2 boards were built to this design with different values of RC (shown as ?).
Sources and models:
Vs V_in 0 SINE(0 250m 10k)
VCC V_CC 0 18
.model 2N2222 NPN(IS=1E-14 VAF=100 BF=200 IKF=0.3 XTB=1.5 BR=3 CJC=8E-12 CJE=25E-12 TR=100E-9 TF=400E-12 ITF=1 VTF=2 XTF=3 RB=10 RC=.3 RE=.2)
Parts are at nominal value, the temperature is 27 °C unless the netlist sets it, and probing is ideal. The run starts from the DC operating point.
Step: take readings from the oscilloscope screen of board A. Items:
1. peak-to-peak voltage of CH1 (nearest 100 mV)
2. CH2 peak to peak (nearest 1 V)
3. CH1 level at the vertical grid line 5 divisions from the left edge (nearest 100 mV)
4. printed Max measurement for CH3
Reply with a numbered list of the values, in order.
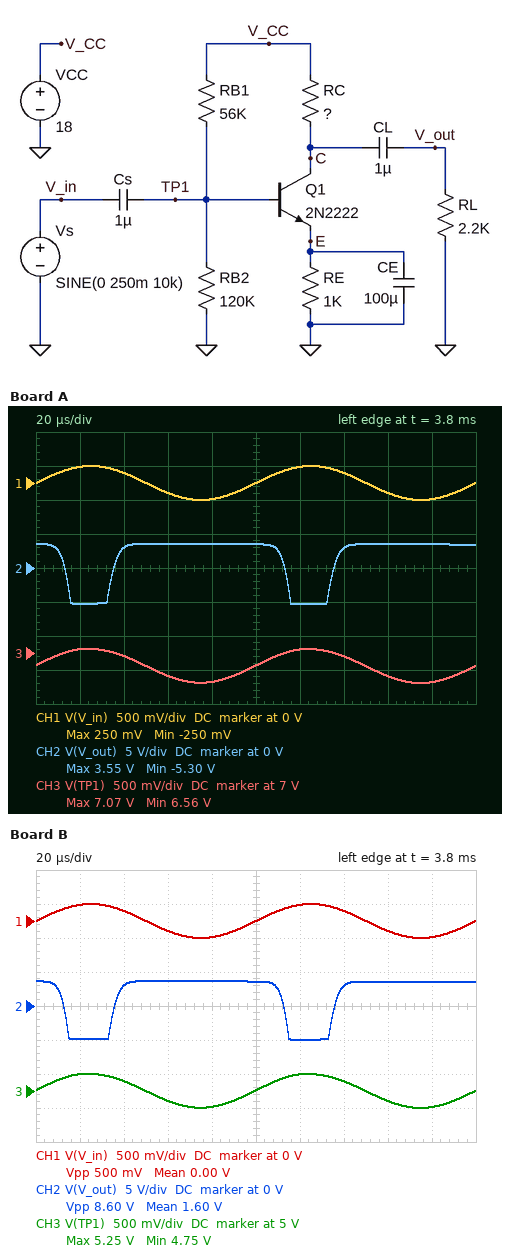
1. 500 mV
2. 9 V
3. 0 V
4. 7.07 V
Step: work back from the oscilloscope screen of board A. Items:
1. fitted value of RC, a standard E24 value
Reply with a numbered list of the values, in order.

1. 1.8 kΩ
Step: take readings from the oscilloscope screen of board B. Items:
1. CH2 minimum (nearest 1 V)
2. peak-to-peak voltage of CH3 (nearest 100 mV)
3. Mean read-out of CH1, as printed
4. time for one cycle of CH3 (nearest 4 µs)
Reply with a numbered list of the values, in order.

1. -5 V
2. 500 mV
3. 0.00 V
4. 100 µs
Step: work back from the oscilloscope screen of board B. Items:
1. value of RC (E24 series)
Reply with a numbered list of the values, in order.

1. 3 kΩ
